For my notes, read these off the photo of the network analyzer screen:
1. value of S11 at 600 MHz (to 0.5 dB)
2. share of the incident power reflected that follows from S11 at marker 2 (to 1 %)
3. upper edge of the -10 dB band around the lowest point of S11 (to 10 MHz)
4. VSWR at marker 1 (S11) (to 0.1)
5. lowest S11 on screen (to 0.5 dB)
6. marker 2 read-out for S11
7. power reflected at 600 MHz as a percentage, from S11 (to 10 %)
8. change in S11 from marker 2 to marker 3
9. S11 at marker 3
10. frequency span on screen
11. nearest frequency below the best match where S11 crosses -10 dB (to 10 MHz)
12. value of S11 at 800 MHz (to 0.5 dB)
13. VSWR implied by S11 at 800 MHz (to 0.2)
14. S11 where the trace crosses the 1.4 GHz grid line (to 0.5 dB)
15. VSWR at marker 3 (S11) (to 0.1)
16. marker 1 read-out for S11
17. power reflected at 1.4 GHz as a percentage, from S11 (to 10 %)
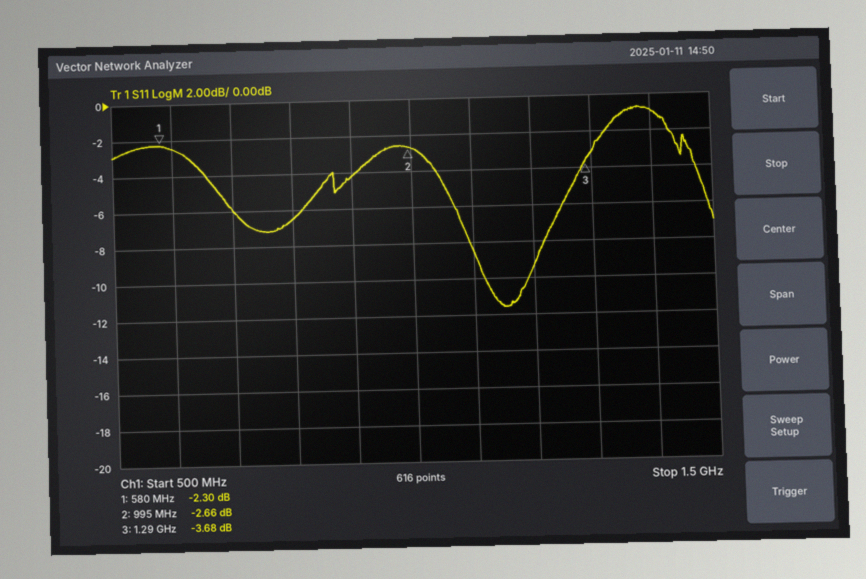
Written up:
-2.5 dB
54 %
1.19 GHz
7.6
-11.5 dB
-2.66 dB
60 %
-1.02 dB
-3.68 dB
1 GHz
1.12 GHz
-6.5 dB
2.8
-1.0 dB
4.8
-2.30 dB
80 %
